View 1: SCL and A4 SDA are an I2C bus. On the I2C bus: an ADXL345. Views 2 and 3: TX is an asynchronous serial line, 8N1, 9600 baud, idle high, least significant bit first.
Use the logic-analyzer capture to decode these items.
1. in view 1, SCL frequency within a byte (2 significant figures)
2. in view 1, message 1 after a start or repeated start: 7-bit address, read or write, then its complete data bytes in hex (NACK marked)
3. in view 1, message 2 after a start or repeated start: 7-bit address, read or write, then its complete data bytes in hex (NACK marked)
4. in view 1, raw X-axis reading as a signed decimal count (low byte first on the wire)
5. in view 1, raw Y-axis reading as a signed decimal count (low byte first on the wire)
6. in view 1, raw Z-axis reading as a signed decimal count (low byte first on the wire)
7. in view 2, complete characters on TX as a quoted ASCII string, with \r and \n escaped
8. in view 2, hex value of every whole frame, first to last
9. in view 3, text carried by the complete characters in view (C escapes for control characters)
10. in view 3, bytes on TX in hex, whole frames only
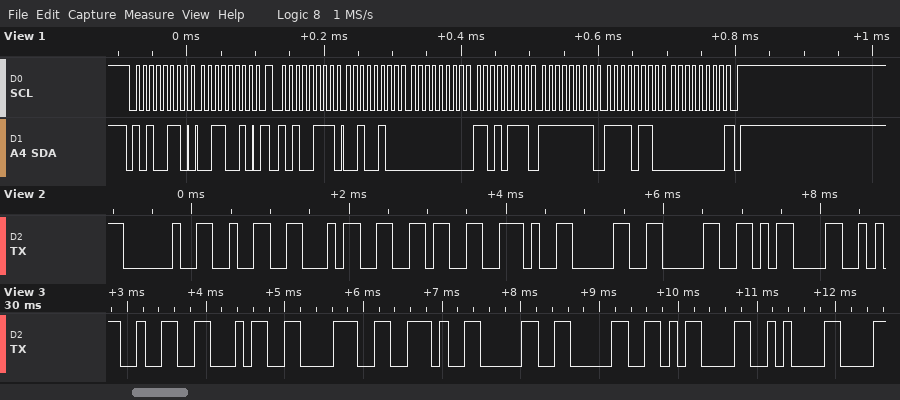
100 kHz
0x53 write: 32
0x53 read: 24 00 D7 FF F6 00 NACK
36
-41
246
" 246.00\r"
20 32 34 36 2E 30 30 0D
"248.00\r\n"
0x32 0x34 0x38 0x2E 0x30 0x30 0x0D 0x0A
